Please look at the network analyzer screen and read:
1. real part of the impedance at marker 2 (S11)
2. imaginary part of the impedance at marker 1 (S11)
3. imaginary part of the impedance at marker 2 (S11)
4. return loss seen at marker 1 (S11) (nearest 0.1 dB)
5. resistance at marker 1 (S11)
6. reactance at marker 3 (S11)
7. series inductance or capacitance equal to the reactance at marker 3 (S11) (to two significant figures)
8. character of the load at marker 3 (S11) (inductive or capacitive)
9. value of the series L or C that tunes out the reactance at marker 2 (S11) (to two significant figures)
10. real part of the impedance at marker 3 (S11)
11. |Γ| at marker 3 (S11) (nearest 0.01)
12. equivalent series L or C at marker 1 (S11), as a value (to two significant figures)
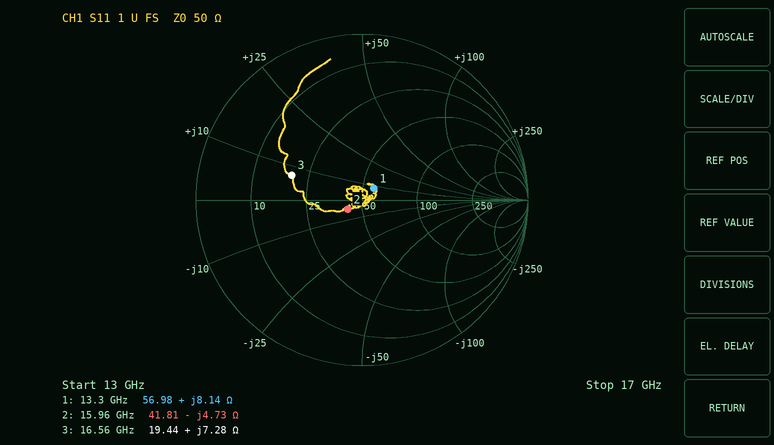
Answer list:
41.81 Ω
+8.14 Ω
-4.73 Ω
20.0 dB
56.98 Ω
+7.28 Ω
70 pH
inductive
47 pH
19.44 Ω
0.45
97 pH
